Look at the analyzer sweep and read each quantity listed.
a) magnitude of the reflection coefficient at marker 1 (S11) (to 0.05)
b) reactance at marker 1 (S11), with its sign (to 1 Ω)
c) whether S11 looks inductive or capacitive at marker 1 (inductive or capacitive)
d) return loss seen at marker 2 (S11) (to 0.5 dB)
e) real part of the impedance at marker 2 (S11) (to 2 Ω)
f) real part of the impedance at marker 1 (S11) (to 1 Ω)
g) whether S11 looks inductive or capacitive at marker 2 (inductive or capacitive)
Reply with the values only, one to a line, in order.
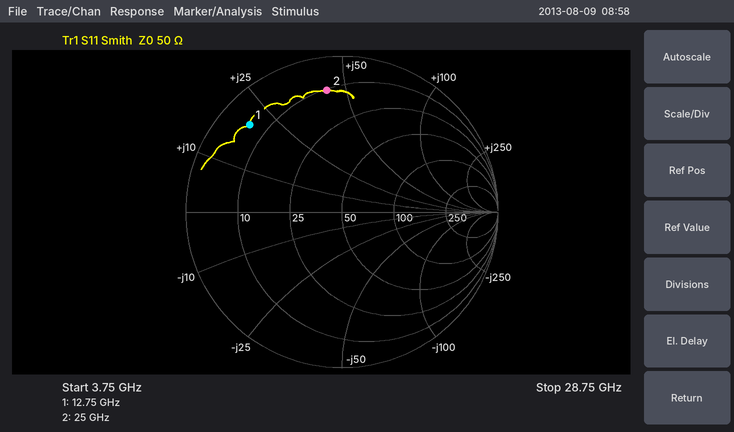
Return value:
0.80
+20 Ω
inductive
2.0 dB
10 Ω
6 Ω
inductive
